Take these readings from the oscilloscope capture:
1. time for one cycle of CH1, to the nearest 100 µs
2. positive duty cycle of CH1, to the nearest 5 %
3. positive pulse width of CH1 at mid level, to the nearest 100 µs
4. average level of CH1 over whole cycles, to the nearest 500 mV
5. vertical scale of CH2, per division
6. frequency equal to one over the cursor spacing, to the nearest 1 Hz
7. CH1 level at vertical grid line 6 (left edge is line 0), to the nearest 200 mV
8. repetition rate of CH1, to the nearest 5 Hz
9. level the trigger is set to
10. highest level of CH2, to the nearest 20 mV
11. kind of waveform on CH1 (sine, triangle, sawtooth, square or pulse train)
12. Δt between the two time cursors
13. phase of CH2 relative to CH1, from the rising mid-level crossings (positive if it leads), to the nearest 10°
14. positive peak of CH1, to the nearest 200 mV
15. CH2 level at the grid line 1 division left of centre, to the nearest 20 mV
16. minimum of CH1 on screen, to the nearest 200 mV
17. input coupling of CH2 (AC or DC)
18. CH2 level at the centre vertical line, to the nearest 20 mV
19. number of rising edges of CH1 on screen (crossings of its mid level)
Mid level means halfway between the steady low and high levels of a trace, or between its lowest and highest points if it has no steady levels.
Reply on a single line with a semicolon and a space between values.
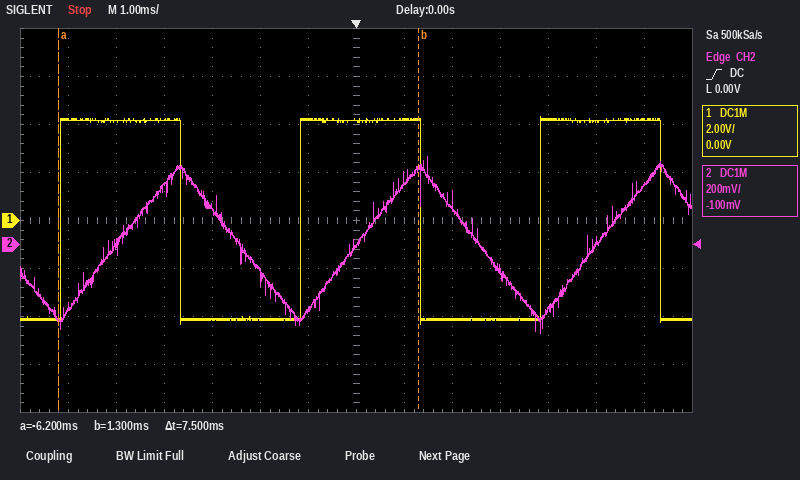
5.0 ms; 50 %; 2.5 ms; 0.0 V; 200 mV; 133 Hz; 4.2 V; 200 Hz; 0.00 V; 360 mV; square; 7.5 ms; -80°; 4.4 V; -280 mV; -4.4 V; DC; 0 mV; 3
